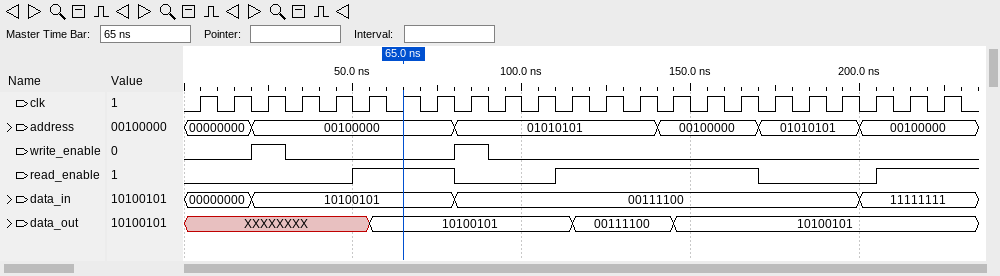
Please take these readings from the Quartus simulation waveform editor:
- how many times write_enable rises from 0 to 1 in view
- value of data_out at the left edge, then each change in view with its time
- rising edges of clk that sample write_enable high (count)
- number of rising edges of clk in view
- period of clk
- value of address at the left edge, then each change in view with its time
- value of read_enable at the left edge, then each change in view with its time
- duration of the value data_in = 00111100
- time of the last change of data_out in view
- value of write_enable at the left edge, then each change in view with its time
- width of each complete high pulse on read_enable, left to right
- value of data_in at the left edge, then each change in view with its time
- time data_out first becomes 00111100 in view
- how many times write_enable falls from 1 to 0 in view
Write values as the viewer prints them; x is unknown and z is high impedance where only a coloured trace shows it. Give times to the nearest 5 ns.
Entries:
2
XXXXXXXX, 10100101 at 55 ns, 00111100 at 115 ns, 10100101 at 145 ns
2
23
10 ns
00000000, 00100000 at 20 ns, 01010101 at 80 ns, 00100000 at 140 ns, 01010101 at 170 ns, 00100000 at 200 ns
0, 1 at 50 ns, 0 at 80 ns, 1 at 110 ns, 0 at 170 ns, 1 at 205 ns
120 ns
145 ns
0, 1 at 20 ns, 0 at 30 ns, 1 at 80 ns, 0 at 90 ns
30 ns, 60 ns
00000000, 10100101 at 20 ns, 00111100 at 80 ns, 11111111 at 200 ns
115 ns
2
